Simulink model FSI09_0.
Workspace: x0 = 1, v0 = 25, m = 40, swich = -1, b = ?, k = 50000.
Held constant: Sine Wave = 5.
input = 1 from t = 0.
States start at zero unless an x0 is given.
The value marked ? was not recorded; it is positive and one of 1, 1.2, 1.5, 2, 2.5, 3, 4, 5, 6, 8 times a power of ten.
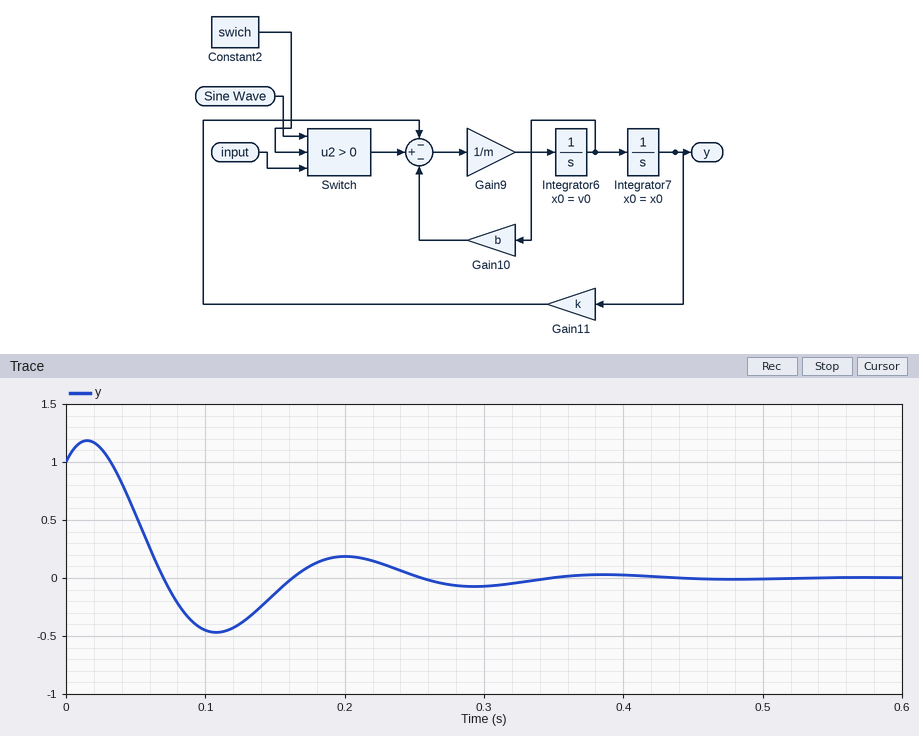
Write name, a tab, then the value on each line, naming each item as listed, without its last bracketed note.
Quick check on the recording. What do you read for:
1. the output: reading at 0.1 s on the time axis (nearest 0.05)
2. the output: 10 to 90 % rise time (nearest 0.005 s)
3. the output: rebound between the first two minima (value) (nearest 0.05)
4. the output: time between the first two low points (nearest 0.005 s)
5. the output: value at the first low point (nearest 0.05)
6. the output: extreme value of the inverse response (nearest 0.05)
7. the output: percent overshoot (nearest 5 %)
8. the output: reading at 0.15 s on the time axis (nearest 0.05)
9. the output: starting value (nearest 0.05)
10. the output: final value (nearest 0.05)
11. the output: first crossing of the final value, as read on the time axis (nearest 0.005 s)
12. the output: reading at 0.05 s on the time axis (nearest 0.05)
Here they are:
the output: reading at 0.1 s on the time axis	-0.45
the output: 10 to 90 % rise time	0.030 s
the output: rebound between the first two minima (value)	0.20
the output: time between the first two low points	0.185 s
the output: value at the first low point	-0.45
the output: extreme value of the inverse response	1.20
the output: percent overshoot	45 %
the output: reading at 0.15 s on the time axis	-0.15
the output: starting value	1.00
the output: final value	0.00
the output: first crossing of the final value, as read on the time axis	0.070 s
the output: reading at 0.05 s on the time axis	0.55
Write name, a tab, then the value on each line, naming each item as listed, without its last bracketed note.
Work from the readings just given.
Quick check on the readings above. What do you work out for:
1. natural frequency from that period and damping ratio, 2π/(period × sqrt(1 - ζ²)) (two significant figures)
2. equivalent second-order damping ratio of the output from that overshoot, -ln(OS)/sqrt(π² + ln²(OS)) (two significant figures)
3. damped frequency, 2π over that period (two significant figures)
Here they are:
natural frequency from that period and damping ratio, 2π/(period × sqrt(1 - ζ²))	35 rad/s
equivalent second-order damping ratio of the output from that overshoot, -ln(OS)/sqrt(π² + ln²(OS))	0.25
damped frequency, 2π over that period	34 rad/s
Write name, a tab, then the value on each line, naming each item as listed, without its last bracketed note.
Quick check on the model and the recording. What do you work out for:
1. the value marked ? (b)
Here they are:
the value marked ?	800
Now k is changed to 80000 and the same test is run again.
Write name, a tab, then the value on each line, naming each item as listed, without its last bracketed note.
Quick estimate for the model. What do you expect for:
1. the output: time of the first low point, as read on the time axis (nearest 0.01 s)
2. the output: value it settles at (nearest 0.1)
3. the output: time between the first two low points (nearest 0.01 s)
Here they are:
the output: time of the first low point, as read on the time axis	0.08 s
the output: value it settles at	0.0
the output: time between the first two low points	0.14 s
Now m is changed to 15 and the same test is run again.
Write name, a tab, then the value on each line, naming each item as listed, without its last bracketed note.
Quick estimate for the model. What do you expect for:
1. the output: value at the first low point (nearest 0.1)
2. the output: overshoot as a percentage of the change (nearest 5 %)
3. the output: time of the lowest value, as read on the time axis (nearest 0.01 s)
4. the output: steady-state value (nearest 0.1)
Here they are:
the output: value at the first low point	-0.2
the output: overshoot as a percentage of the change	20 %
the output: time of the lowest value, as read on the time axis	0.07 s
the output: steady-state value	0.0
